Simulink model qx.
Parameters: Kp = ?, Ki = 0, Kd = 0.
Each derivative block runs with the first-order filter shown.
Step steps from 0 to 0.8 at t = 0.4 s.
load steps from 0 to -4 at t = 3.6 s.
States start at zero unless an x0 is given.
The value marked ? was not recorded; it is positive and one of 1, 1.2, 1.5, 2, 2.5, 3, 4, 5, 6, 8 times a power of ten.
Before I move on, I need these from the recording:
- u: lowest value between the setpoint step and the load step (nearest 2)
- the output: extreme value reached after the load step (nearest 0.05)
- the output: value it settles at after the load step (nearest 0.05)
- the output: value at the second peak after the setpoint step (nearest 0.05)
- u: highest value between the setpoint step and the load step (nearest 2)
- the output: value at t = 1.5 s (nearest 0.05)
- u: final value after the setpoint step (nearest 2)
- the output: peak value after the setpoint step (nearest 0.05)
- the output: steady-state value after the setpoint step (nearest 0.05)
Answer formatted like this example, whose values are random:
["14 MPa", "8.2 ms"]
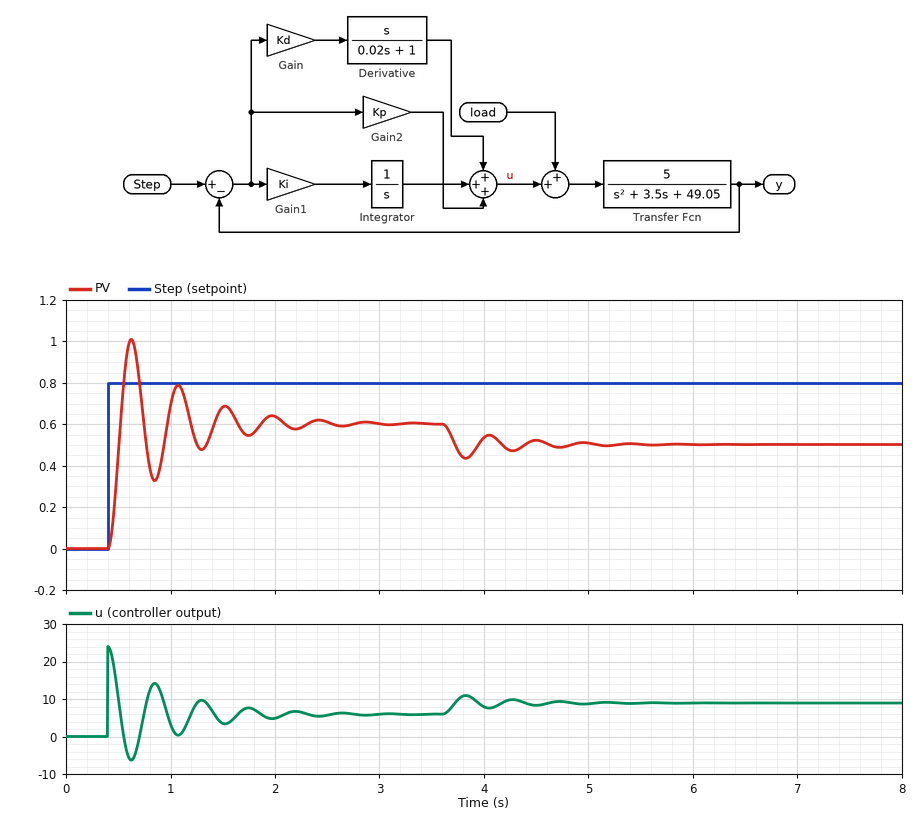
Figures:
["-6", "0.45", "0.50", "0.80", "24", "0.70", "6", "1.00", "0.60"]
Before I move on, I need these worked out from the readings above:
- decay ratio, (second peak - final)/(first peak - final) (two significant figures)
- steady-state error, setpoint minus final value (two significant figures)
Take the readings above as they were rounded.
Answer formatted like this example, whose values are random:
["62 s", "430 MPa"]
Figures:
["0.50", "0.20"]
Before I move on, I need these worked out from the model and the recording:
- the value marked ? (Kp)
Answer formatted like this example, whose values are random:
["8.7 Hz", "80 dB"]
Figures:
["30"]
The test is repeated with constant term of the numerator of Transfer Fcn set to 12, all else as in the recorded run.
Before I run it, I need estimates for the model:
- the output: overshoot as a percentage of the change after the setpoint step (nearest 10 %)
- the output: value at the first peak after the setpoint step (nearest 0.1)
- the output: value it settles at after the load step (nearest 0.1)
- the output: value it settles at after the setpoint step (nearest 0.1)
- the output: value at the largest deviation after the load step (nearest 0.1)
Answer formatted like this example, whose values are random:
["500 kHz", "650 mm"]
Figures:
["80 %", "1.2", "0.6", "0.7", "0.5"]
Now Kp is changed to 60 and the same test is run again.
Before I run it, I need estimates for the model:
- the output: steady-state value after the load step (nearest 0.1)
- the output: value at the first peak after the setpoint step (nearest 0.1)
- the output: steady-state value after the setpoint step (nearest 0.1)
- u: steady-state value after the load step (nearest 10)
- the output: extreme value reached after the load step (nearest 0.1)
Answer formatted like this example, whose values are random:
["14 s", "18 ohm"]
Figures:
["0.6", "1.2", "0.7", "10", "0.6"]
